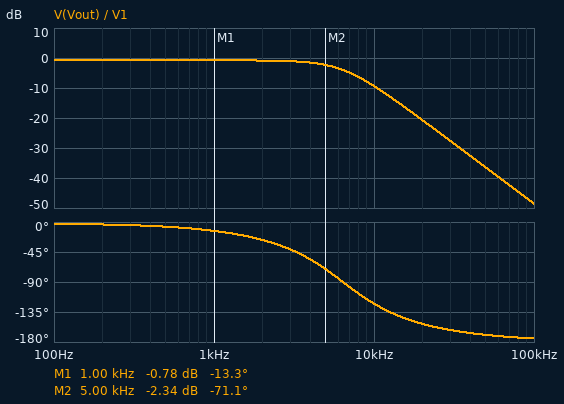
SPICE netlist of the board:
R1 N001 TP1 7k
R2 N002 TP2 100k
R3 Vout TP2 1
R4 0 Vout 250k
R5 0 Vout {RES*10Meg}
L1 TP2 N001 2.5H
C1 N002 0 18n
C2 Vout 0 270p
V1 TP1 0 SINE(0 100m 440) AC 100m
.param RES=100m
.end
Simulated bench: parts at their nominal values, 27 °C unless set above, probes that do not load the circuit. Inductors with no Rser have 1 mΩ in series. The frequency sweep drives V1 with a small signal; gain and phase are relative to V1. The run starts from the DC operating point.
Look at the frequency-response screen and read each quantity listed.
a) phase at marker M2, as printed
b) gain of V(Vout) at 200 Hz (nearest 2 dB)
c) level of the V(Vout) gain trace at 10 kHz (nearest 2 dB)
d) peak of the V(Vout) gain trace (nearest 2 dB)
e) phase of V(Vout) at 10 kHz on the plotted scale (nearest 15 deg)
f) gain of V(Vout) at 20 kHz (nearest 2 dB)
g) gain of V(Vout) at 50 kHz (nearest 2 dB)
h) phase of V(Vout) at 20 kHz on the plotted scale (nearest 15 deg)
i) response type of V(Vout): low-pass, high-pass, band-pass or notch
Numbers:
-71.1 deg
0 dB
-10 dB
0 dB
-120 deg
-20 dB
-36 dB
-150 deg
low-pass
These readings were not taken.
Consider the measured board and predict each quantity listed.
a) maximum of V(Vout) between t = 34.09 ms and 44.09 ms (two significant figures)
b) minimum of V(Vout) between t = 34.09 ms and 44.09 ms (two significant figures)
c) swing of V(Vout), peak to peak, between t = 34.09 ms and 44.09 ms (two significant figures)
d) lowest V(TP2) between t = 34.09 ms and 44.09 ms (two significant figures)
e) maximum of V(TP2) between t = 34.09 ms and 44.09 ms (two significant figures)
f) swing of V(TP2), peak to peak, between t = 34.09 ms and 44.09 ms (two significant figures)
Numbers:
92 mV
-92 mV
180 mV
-92 mV
92 mV
180 mV
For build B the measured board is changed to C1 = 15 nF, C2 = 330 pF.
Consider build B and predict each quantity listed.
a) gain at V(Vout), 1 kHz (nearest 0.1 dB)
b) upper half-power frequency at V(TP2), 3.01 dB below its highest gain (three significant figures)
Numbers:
-0.7 dB
5.85 kHz
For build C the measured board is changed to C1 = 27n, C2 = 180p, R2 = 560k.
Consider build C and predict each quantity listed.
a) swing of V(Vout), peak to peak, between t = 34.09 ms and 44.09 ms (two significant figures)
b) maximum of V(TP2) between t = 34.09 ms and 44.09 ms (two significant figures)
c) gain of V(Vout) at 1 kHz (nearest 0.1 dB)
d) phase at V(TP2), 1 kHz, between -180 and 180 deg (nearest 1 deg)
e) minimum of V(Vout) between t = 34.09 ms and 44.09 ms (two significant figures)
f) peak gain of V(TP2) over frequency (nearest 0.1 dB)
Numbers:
190 mV
96 mV
-0.3 dB
-6 deg
-96 mV
2.0 dB
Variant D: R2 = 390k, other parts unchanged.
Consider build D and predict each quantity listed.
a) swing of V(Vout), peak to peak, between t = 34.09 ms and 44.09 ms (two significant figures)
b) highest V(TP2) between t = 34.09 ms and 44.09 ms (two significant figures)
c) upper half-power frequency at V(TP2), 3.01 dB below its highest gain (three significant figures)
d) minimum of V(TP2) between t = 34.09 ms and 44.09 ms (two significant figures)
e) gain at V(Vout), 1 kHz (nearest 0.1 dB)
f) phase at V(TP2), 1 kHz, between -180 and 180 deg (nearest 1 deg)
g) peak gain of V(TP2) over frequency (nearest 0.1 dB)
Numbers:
190 mV
95 mV
7.47 kHz
-95 mV
-0.3 dB
-7 deg
2.4 dB
